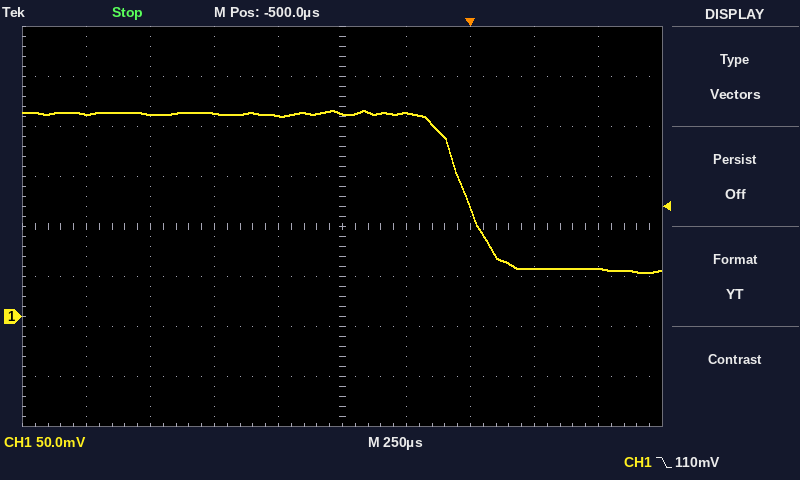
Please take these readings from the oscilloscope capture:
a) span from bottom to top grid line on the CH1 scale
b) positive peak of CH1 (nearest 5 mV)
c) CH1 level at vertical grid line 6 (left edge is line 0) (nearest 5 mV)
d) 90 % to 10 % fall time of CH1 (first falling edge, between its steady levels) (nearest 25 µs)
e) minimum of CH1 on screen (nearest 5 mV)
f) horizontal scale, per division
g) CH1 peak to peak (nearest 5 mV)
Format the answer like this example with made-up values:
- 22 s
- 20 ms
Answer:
- 400 mV
- 205 mV
- 205 mV
- 225 µs
- 45 mV
- 250 µs
- 160 mV
